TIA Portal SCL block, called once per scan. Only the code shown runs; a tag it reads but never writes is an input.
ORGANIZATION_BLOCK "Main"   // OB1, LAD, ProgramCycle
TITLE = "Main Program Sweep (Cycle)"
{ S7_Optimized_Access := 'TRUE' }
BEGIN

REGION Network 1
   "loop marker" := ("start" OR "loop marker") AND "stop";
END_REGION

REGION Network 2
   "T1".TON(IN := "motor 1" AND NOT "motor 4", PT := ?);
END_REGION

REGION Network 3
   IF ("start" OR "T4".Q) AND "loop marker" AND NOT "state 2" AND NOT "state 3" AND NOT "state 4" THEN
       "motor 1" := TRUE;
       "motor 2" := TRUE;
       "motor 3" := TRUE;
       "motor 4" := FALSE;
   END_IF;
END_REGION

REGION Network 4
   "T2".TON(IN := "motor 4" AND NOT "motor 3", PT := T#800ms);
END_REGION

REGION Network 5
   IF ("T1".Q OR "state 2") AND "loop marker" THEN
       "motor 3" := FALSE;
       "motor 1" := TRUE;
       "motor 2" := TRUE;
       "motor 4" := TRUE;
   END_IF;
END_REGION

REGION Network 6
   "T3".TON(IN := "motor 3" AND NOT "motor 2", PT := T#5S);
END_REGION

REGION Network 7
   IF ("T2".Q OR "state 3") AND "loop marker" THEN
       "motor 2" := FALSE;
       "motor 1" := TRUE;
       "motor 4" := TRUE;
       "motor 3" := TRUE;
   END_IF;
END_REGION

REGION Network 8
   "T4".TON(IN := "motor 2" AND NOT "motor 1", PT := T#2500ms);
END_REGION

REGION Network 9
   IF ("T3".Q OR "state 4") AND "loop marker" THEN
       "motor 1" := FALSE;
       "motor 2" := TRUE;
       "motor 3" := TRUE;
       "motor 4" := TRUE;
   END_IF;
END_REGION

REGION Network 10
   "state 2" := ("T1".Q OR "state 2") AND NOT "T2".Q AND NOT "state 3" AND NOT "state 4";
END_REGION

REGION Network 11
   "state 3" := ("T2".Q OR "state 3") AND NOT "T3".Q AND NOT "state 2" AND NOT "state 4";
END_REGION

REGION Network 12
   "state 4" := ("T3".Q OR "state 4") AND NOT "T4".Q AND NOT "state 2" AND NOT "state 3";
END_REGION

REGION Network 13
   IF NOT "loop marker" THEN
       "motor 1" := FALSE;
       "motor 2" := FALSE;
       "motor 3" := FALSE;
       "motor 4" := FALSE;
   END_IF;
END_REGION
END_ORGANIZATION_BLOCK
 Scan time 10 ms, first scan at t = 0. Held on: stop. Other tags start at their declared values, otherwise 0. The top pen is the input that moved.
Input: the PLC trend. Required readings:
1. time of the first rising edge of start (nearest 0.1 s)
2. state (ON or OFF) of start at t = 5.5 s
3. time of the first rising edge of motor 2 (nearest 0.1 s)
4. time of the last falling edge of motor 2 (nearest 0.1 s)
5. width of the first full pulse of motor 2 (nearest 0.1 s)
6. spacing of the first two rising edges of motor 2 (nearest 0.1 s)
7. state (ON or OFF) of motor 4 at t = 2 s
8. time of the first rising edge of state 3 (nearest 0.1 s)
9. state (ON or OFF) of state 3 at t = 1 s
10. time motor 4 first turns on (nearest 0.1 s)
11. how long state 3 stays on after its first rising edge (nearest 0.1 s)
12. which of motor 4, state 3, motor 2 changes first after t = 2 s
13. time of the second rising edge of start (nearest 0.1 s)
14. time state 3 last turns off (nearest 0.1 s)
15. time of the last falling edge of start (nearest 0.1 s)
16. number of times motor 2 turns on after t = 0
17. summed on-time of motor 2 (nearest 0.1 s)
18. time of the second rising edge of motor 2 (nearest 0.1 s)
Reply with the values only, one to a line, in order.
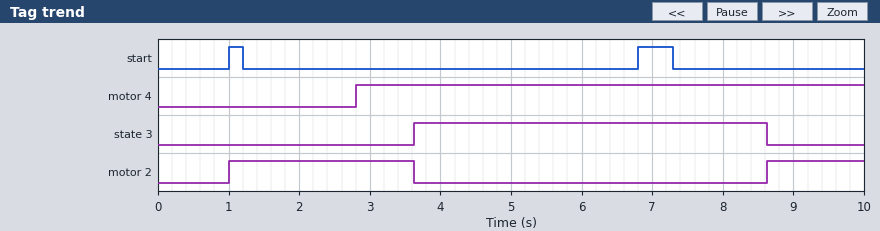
1.0 s
OFF
1.0 s
3.6 s
2.6 s
7.6 s
OFF
3.6 s
OFF
2.8 s
5.0 s
motor 4
6.8 s
8.6 s
7.3 s
2
4.0 s
8.6 s
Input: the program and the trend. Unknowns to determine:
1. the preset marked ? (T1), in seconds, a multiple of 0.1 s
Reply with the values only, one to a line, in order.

1.8 s
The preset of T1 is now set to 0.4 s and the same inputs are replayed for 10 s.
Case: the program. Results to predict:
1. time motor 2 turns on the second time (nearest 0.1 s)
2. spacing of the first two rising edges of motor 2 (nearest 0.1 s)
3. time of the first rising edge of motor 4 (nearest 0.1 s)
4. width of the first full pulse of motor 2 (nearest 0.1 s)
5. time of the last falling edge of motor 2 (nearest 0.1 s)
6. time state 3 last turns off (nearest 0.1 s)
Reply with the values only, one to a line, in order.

7.2 s
6.2 s
1.4 s
1.2 s
2.2 s
7.2 s
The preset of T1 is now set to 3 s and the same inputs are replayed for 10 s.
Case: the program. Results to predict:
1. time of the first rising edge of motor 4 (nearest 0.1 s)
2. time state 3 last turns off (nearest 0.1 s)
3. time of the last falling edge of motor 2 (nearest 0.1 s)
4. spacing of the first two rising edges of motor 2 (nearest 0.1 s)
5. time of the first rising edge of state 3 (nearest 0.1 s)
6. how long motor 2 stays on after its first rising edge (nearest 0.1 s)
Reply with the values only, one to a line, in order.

4.0 s
9.8 s
4.8 s
8.8 s
4.8 s
3.8 s
